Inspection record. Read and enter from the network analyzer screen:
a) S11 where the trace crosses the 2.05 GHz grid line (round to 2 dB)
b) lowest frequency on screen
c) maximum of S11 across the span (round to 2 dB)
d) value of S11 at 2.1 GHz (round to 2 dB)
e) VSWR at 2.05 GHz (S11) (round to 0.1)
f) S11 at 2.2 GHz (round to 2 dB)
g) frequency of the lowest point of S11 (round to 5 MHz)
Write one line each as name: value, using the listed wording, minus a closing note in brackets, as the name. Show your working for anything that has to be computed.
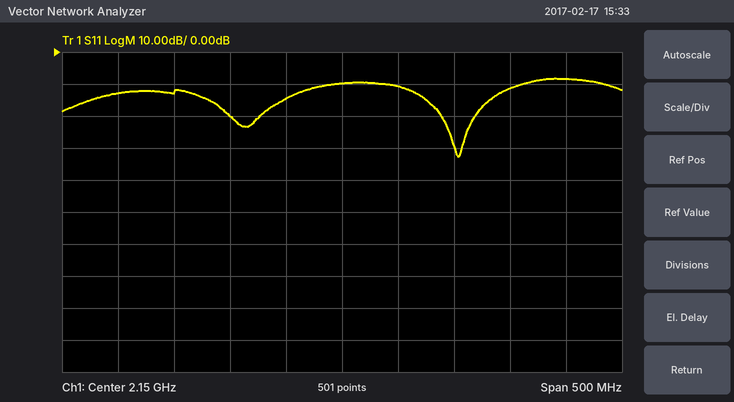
S11 where the trace crosses the 2.05 GHz grid line: -20 dB
lowest frequency on screen: 1.9 GHz
maximum of S11 across the span: -8 dB
value of S11 at 2.1 GHz: -14 dB
VSWR at 2.05 GHz (S11): |Γ| = 10^(-20/20) = 0.1000; VSWR = (1 + 0.1000)/(1 − 0.1000) ≈ 1.2
S11 at 2.2 GHz: -10 dB
frequency of the lowest point of S11: 2.255 GHz
